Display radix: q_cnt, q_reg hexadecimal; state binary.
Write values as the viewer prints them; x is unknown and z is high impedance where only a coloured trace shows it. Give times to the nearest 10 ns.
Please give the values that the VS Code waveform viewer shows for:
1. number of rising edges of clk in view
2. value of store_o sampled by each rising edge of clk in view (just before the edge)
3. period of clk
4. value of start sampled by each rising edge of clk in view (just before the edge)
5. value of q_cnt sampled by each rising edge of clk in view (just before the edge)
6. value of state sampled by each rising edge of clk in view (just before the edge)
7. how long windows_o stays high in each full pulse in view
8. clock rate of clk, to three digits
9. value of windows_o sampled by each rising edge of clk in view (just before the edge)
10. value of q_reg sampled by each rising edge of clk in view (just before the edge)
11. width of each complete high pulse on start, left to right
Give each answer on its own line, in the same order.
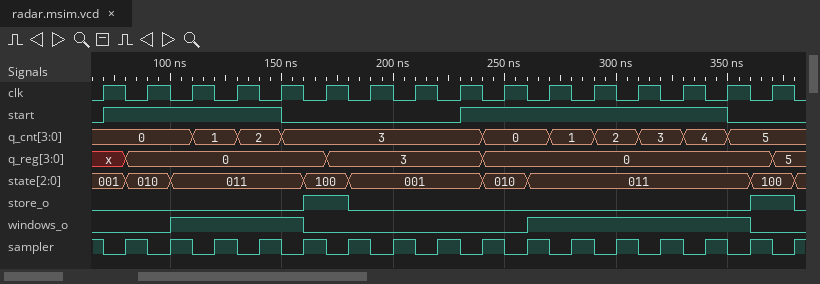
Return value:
16
0 0 0 0 0 1 0 0 0 0 0 0 0 0 0 1
20 ns
0 1 1 1 1 0 0 0 0 1 1 1 1 1 1 0
0, 0, 0, 1, 2, 3, 3, 3, 3, 0, 0, 1, 2, 3, 4, 5
001, 010, 011, 011, 011, 100, 001, 001, 001, 010, 011, 011, 011, 011, 011, 100
60 ns, 100 ns
50.0 MHz
0 0 1 1 1 0 0 0 0 0 1 1 1 1 1 0
x, 0, 0, 0, 0, 0, 3, 3, 3, 0, 0, 0, 0, 0, 0, 0
80 ns, 120 ns
